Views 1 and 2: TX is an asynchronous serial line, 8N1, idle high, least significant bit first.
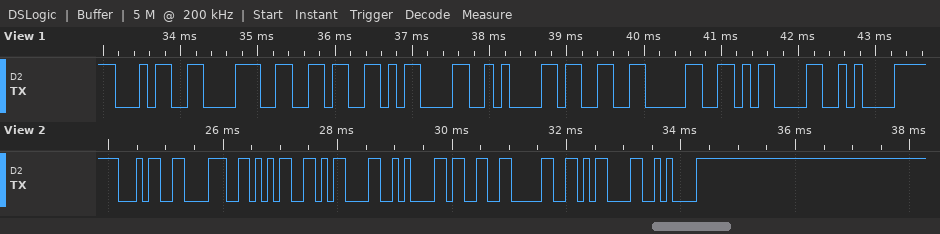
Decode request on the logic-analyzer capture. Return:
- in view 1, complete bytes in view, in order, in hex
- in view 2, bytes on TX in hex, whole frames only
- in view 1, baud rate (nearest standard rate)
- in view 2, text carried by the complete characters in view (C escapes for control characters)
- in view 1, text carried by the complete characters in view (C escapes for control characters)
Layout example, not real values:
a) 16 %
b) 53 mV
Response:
a) 34 38 36 0D 0A 33 30 0D 0A
b) 34 38 35 0D 0A 33 30 0D 0A
c) 9600 baud
d) "485\r\n30\r\n"
e) "486\r\n30\r\n"
